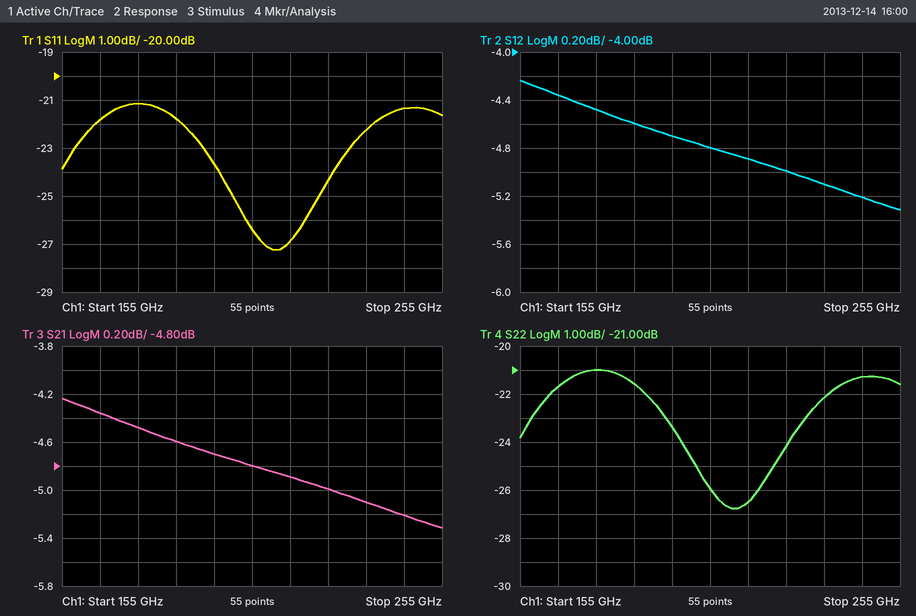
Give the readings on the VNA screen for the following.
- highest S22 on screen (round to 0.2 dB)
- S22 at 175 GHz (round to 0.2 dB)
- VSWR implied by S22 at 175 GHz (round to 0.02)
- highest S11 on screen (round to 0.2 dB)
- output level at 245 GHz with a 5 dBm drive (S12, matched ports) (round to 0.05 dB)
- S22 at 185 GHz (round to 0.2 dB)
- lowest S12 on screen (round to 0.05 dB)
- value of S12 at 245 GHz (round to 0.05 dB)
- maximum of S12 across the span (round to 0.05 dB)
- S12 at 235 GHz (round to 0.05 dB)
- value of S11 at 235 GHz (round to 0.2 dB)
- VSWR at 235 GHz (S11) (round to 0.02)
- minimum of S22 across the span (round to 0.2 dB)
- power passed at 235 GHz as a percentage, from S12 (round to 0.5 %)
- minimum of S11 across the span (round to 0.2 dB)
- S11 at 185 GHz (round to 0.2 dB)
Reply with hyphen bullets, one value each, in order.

- -21.0 dB
- -21.0 dB
- 1.20
- -21.2 dB
- -0.20 dBm
- -21.6 dB
- -5.30 dB
- -5.20 dB
- -4.25 dB
- -5.10 dB
- -22.2 dB
- 1.16
- -26.8 dB
- 31.0 %
- -27.2 dB
- -21.8 dB
